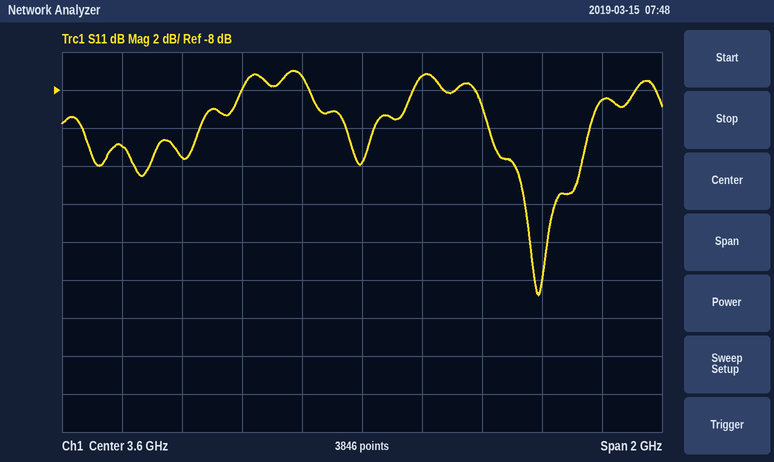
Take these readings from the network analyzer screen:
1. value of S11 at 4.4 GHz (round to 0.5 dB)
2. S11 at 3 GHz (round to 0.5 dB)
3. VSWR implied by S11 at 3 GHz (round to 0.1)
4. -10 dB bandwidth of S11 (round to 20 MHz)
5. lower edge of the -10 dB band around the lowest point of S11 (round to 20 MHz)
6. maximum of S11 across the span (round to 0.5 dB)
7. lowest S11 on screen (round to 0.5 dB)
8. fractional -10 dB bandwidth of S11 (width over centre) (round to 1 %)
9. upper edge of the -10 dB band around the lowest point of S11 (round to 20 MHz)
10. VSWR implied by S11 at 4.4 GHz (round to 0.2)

-8.5 dB
-11.5 dB
1.7
340 MHz
4.02 GHz
-7.0 dB
-19.0 dB
8 %
4.36 GHz
2.2
